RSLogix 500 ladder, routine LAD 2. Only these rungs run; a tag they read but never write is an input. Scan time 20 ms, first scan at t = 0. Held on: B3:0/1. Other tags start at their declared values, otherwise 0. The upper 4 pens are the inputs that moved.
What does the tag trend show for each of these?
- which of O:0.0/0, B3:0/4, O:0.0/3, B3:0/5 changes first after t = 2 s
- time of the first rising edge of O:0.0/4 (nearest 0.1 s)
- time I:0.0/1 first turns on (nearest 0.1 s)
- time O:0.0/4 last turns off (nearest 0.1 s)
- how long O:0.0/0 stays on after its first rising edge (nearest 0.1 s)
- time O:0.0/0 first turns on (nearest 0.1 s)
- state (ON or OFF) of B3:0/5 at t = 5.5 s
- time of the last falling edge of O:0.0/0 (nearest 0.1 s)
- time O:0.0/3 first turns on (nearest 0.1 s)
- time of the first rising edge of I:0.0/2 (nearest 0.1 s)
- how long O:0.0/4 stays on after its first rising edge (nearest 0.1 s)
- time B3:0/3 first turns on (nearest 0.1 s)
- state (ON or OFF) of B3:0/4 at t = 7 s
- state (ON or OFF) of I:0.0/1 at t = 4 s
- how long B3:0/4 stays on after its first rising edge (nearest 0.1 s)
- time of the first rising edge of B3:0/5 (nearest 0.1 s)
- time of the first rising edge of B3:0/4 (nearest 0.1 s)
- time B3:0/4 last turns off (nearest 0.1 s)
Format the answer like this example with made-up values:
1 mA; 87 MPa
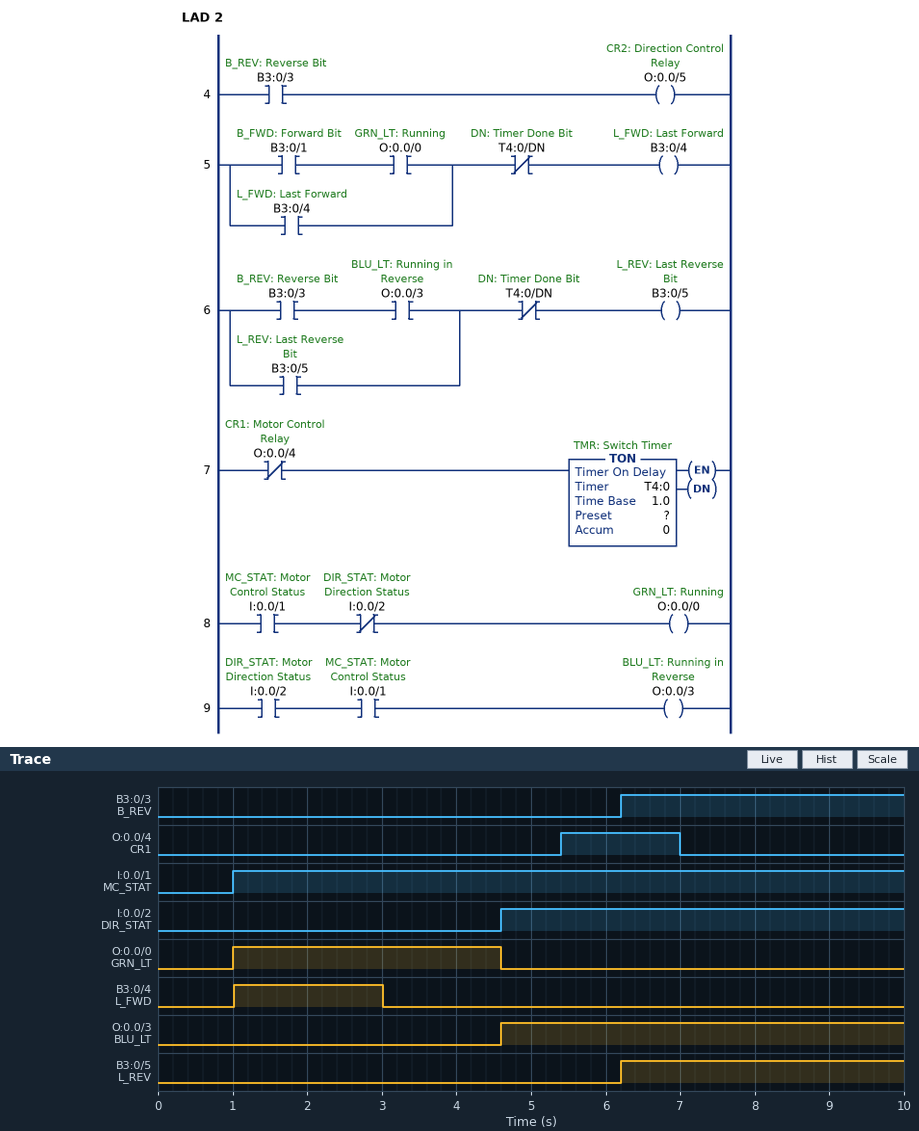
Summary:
B3:0/4; 5.4 s; 1.0 s; 7.0 s; 3.6 s; 1.0 s; OFF; 4.6 s; 4.6 s; 4.6 s; 1.6 s; 6.2 s; OFF; ON; 2.0 s; 6.2 s; 1.0 s; 3.0 s
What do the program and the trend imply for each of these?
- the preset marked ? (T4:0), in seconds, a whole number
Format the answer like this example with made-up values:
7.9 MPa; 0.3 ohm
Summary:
3 s
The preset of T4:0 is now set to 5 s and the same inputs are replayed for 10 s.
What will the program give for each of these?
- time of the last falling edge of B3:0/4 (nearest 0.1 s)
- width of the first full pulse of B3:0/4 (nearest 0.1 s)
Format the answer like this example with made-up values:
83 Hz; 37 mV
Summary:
5.0 s; 4.0 s
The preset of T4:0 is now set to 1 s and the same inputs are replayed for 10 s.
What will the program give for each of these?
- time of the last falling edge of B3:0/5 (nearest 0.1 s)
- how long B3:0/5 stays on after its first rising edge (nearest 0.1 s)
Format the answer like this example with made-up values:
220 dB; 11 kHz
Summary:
8.0 s; 1.8 s
